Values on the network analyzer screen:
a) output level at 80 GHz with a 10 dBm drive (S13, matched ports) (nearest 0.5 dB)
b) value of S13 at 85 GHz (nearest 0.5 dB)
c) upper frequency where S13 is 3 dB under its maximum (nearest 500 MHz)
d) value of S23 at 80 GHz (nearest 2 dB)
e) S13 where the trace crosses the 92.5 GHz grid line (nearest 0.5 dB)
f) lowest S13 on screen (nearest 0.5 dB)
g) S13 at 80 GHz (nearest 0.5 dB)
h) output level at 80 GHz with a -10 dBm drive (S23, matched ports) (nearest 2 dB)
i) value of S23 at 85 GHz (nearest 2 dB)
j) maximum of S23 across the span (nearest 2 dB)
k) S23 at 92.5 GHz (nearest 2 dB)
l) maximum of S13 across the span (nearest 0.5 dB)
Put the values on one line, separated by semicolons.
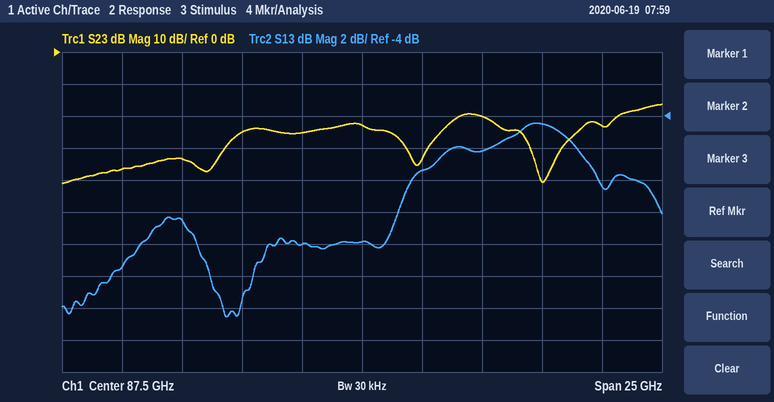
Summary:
-0.5 dBm; -12.0 dB; 97.0 GHz; -34 dB; -6.0 dB; -16.5 dB; -10.5 dB; -44 dBm; -26 dB; -16 dB; -20 dB; -4.5 dB
